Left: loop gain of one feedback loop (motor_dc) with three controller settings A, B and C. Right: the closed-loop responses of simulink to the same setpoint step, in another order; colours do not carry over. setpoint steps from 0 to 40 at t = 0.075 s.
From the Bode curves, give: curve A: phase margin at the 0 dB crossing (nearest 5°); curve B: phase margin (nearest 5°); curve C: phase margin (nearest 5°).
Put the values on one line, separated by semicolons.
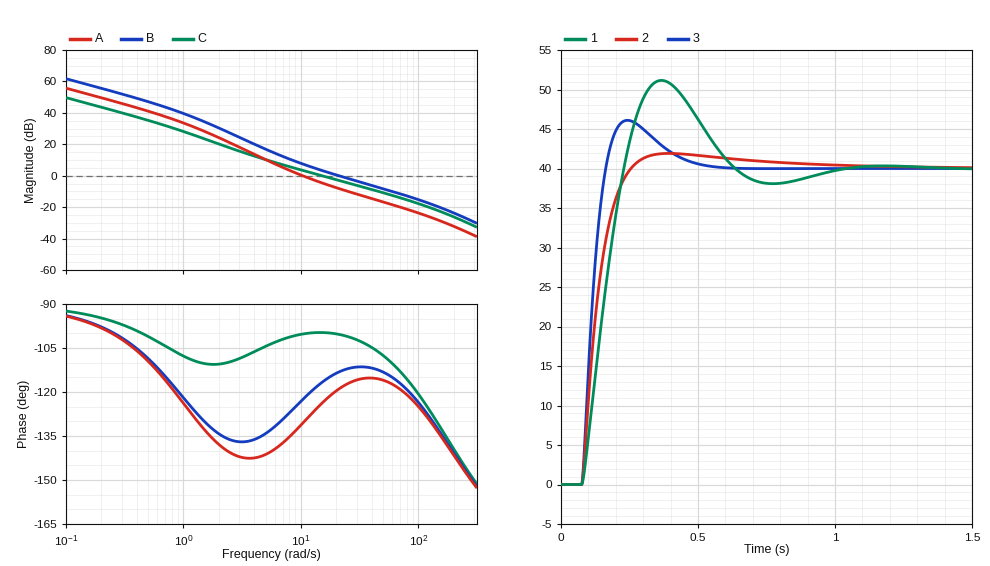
50°; 65°; 80°
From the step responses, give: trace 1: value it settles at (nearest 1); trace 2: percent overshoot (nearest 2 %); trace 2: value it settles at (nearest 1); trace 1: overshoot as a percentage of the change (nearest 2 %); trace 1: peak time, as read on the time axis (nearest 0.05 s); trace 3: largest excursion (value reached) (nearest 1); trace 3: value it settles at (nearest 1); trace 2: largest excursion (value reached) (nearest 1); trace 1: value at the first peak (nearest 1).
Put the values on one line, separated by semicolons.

40; 4 %; 40; 28 %; 0.35 s; 46; 40; 42; 51
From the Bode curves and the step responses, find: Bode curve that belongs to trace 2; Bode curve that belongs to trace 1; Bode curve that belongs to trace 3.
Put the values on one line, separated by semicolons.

C; A; B
